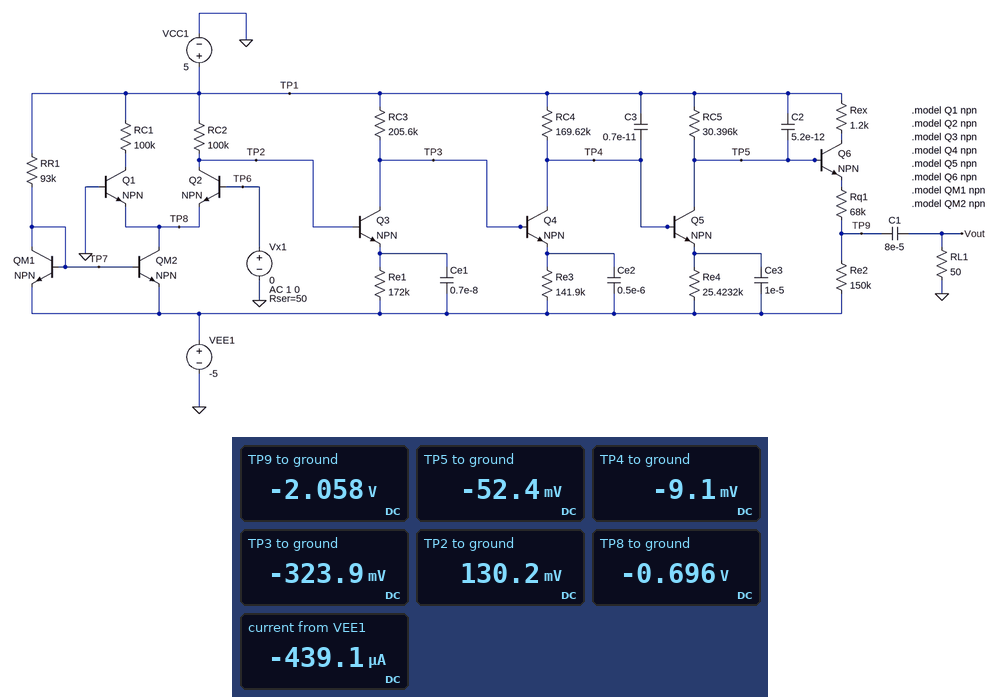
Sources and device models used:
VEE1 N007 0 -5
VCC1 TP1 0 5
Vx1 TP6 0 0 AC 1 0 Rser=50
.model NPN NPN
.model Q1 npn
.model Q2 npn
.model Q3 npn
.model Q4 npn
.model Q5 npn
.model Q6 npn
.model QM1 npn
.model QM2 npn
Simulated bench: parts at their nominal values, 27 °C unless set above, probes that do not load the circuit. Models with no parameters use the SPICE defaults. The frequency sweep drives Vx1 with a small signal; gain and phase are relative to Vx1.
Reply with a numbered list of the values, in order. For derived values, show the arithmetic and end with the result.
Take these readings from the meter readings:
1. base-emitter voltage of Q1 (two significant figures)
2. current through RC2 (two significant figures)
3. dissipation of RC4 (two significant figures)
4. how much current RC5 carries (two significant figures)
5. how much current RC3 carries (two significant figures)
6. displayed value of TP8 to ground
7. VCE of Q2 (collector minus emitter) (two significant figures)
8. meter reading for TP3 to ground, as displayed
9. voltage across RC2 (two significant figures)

1. 0 V - (-696 mV) = 700 mV
2. (5 V - 130.2 mV) / 100 kΩ = 49 µA
3. (5 V - (-9.1 mV))^2 / 169.6 kΩ = 150 µW
4. (5 V - (-52.4 mV)) / 30.4 kΩ = 170 µA
5. (5 V - (-323.9 mV)) / 205.6 kΩ = 26 µA
6. -0.696 V
7. 130.2 mV - (-696 mV) = 830 mV
8. -323.9 mV
9. 5 V - 130.2 mV = 4.9 V
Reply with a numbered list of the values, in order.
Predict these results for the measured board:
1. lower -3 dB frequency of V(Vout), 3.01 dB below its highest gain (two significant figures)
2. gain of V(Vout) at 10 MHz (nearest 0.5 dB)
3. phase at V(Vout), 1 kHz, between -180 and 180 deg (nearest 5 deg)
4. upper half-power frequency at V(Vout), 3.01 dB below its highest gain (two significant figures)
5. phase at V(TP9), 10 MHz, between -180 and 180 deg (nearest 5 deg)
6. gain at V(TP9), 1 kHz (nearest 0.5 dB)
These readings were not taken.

1. 7.7 kHz
2. 36.5 dB
3. 80 deg
4. 800 kHz
5. -165 deg
6. 54.5 dB
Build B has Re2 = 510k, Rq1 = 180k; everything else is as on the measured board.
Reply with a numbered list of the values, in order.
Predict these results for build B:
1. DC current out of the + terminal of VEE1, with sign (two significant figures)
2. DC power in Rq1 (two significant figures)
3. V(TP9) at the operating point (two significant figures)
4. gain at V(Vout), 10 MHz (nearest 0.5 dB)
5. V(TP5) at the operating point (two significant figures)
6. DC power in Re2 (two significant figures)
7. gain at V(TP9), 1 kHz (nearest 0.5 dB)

1. -430 µA
2. 7.0 µW
3. -1.8 V
4. 28.0 dB
5. -48 mV
6. 20 µW
7. 46.0 dB
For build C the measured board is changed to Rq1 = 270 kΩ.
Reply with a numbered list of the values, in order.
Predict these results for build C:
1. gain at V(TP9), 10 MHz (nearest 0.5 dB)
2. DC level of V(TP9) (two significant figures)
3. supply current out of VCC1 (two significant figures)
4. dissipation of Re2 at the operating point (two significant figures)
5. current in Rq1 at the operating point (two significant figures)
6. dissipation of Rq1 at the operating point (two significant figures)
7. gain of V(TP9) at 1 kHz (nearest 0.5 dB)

1. 24.5 dB
2. -3.5 V
3. 430 µA
4. 16 µW
5. 10 µA
6. 28 µW
7. 42.5 dB
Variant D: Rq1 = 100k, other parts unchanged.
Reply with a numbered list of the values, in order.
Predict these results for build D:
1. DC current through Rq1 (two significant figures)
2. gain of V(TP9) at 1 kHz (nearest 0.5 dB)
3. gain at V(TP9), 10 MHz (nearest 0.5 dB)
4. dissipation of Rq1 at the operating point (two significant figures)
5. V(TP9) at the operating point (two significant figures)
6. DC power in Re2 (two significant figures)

1. 17 µA
2. 51.0 dB
3. 33.0 dB
4. 29 µW
5. -2.4 V
6. 44 µW
